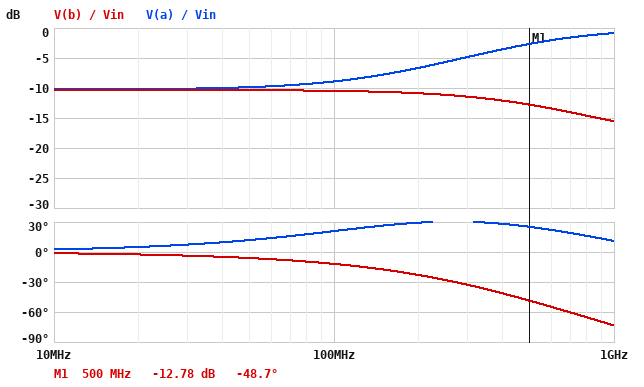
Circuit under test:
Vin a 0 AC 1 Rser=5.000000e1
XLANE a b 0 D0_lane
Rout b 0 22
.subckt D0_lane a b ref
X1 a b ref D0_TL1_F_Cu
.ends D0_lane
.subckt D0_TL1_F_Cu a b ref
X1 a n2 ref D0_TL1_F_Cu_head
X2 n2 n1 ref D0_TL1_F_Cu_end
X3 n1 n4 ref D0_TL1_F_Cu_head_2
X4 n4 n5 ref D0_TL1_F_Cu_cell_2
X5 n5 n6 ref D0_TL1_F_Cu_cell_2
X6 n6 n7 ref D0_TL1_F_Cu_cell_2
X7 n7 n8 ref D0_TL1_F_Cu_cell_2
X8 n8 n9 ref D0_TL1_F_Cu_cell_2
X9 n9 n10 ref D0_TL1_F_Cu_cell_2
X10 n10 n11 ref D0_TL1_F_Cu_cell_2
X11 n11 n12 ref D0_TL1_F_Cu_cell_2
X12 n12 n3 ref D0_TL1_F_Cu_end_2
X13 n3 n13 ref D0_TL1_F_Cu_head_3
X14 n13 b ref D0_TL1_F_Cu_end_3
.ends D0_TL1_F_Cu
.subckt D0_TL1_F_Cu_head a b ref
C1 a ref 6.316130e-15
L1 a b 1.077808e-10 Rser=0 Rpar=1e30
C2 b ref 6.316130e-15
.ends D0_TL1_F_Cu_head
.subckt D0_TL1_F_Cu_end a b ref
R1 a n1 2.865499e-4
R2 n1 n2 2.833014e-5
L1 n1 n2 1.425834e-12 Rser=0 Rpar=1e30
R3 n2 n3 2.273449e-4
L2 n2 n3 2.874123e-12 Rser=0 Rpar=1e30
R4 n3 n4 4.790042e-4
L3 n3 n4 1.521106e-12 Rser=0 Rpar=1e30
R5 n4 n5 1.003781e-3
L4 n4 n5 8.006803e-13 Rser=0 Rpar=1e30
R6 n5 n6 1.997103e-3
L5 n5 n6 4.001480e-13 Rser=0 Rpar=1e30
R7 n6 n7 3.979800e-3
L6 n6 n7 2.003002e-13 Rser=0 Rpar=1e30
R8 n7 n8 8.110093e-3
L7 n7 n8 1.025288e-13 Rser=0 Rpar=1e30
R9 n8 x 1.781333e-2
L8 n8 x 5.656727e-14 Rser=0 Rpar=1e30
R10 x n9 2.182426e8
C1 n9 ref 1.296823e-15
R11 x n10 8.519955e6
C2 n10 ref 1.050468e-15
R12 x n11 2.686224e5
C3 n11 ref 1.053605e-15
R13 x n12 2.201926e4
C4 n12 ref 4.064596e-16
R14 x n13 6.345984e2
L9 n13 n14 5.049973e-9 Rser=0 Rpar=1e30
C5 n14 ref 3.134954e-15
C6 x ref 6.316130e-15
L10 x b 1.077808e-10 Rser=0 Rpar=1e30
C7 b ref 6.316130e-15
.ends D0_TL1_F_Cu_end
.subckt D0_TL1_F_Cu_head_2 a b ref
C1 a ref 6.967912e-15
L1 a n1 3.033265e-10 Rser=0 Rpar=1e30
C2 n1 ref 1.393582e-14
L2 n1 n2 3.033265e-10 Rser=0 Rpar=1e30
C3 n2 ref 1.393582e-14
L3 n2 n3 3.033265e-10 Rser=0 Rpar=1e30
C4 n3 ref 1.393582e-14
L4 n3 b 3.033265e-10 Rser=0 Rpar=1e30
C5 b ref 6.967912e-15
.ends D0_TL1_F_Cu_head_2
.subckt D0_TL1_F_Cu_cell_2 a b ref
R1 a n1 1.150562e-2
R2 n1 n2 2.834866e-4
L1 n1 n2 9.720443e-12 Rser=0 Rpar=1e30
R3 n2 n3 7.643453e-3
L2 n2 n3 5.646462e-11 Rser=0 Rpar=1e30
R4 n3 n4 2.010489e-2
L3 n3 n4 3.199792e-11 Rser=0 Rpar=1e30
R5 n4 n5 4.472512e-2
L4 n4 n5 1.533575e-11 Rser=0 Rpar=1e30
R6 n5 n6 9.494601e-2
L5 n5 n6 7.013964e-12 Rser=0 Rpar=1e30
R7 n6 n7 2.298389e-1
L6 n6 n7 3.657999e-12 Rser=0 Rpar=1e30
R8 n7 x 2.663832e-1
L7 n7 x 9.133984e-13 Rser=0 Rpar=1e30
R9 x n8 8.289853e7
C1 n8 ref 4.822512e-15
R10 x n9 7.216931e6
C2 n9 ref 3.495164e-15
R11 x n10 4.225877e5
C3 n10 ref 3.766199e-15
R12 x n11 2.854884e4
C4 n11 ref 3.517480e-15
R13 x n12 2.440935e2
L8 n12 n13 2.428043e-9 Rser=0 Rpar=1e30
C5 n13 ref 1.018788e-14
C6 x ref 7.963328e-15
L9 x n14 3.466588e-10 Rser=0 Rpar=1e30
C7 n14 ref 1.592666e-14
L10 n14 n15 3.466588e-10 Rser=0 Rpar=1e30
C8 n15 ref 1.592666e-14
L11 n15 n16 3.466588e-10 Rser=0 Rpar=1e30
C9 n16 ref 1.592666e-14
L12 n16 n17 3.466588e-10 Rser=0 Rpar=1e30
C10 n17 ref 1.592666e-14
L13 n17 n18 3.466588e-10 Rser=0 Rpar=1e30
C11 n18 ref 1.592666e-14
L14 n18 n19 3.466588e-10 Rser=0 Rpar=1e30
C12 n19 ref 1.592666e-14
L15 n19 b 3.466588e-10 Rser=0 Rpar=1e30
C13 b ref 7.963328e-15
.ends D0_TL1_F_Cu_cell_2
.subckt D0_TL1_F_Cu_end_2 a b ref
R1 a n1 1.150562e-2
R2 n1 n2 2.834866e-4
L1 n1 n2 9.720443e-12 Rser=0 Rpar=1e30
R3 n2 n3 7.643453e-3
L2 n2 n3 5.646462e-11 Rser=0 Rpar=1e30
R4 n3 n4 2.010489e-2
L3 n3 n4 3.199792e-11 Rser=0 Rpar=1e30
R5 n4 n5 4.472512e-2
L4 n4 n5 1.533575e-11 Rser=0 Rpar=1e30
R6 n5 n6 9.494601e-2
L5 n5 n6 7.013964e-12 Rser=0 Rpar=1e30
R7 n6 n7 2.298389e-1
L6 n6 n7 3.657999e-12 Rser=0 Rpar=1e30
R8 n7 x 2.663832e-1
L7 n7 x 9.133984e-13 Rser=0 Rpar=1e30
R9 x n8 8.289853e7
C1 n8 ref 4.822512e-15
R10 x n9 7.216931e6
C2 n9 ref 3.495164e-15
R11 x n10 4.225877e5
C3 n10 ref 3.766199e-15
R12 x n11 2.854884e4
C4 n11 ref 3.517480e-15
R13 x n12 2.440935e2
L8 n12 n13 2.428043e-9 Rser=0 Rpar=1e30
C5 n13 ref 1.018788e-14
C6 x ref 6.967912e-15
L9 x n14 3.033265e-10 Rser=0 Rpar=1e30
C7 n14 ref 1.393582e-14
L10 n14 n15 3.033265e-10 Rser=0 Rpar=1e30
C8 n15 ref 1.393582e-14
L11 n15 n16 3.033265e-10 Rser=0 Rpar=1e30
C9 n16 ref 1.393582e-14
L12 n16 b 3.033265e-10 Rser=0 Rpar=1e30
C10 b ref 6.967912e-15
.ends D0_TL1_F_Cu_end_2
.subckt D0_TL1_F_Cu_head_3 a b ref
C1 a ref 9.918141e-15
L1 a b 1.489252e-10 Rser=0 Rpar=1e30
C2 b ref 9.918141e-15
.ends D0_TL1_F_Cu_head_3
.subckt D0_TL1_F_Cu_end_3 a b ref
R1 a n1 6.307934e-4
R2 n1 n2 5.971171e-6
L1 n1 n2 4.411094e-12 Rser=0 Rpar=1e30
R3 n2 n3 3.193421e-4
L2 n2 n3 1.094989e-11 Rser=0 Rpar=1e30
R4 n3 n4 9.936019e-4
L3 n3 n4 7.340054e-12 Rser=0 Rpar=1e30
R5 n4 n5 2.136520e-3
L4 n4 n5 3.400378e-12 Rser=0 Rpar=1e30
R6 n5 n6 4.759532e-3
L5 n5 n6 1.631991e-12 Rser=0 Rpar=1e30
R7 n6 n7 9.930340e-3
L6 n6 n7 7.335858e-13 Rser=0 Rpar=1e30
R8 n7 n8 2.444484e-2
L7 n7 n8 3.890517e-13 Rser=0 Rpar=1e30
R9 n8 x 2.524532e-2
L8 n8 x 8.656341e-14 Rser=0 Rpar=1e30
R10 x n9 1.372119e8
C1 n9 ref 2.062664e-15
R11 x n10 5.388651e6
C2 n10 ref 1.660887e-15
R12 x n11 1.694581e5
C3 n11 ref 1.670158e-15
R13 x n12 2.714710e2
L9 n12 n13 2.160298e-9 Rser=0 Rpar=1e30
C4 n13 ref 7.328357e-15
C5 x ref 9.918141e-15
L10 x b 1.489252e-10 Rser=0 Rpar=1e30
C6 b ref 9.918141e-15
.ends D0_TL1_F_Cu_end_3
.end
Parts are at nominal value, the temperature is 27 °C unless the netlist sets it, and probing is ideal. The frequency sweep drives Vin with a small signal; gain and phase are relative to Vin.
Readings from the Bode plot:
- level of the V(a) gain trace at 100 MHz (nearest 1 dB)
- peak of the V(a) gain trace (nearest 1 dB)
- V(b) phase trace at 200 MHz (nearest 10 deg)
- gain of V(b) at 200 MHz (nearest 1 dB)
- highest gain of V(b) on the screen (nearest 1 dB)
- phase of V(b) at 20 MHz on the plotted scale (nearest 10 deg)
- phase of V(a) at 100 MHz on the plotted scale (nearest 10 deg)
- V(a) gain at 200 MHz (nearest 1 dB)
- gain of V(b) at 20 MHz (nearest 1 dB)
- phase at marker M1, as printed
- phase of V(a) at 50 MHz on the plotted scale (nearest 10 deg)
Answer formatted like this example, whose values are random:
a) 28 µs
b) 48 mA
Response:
a) -9 dB
b) -1 dB
c) -20 deg
d) -11 dB
e) -10 dB
f) 0 deg
g) 20 deg
h) -7 dB
i) -10 dB
j) -48.7 deg
k) 10 deg
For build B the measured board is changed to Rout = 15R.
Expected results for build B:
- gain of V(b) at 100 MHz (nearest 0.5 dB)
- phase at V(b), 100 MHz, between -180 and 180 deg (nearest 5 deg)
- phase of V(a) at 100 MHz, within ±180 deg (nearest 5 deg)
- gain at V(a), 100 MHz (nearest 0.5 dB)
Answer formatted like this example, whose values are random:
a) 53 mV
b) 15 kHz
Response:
a) -13.0 dB
b) -15 deg
c) 30 deg
d) -10.0 dB
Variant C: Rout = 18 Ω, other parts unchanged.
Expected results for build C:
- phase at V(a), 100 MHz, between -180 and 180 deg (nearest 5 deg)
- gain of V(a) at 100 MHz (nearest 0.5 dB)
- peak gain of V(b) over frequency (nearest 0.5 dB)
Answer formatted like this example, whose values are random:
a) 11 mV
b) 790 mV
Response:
a) 25 deg
b) -9.5 dB
c) -11.5 dB
